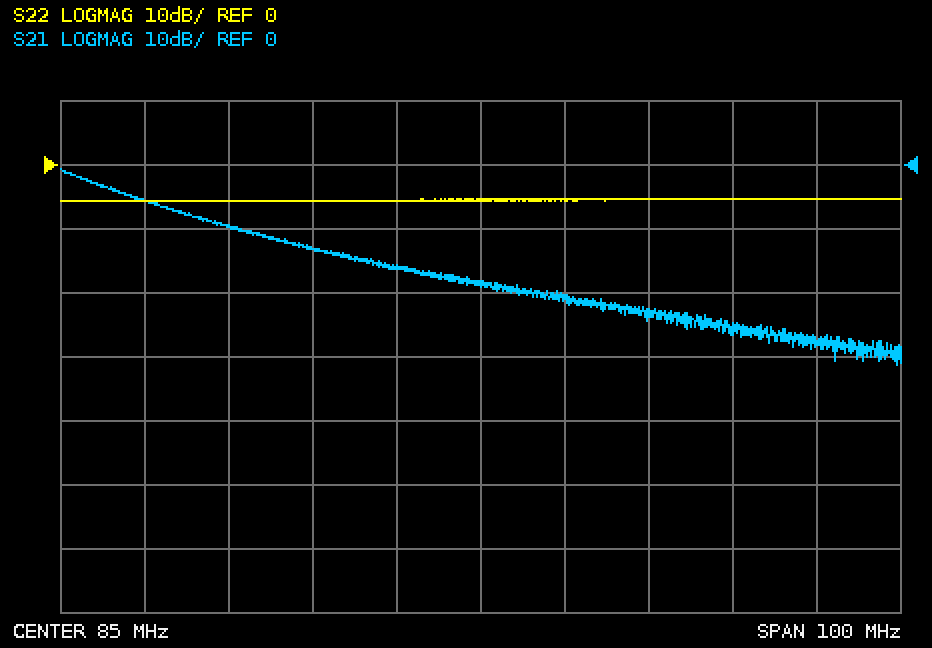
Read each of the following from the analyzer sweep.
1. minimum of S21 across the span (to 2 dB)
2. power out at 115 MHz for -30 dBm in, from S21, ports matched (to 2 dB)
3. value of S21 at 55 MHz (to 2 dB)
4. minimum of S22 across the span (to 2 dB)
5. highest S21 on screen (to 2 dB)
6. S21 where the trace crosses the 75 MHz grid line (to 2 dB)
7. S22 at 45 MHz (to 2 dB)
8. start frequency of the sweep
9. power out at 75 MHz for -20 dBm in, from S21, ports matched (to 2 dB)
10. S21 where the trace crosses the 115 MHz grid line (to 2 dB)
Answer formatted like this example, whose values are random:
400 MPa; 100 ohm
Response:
-32 dB; -56 dBm; -10 dB; -6 dB; 0 dB; -16 dB; -6 dB; 35 MHz; -36 dBm; -26 dB
